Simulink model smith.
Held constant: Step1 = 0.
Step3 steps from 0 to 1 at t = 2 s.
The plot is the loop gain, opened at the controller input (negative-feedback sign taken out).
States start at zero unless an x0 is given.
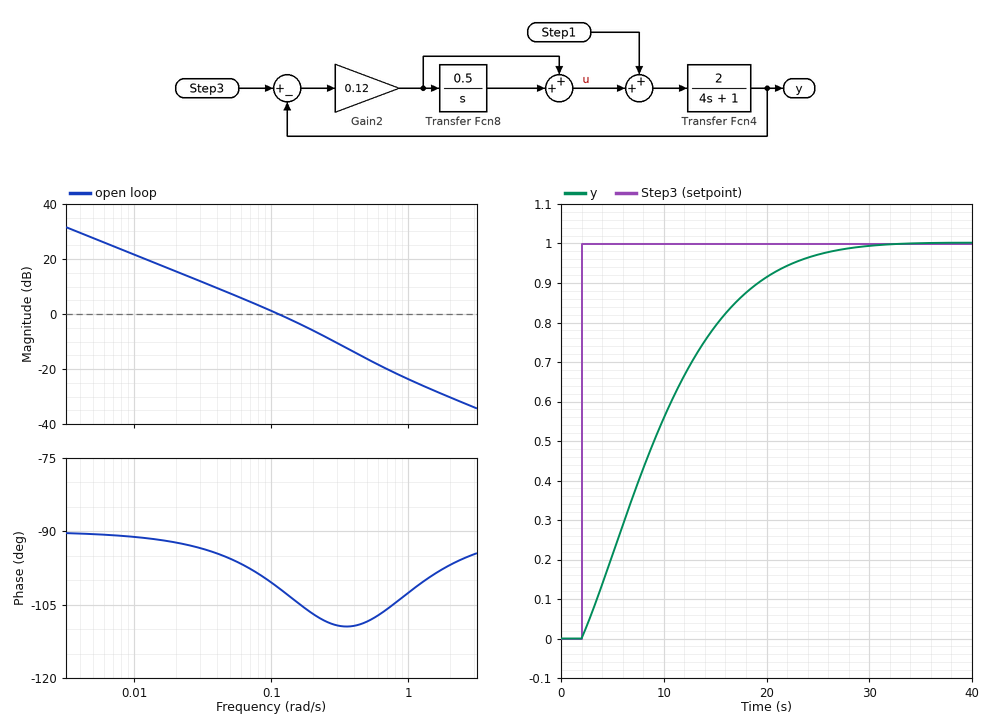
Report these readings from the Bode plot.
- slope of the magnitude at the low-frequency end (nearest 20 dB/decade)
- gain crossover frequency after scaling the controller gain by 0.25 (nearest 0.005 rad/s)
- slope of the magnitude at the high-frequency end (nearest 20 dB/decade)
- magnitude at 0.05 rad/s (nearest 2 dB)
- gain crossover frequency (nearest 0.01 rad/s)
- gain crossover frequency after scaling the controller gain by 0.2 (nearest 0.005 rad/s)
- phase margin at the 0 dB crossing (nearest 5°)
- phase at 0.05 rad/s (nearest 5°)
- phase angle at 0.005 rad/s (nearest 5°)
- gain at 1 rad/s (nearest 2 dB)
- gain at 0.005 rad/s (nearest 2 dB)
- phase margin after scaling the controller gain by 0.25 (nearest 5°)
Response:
-20 dB/decade
0.030 rad/s
-20 dB/decade
8 dB
0.11 rad/s
0.025 rad/s
80°
-95°
-90°
-24 dB
28 dB
85°
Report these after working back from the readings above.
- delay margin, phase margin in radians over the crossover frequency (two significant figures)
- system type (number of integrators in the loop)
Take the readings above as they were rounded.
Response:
13 s
1
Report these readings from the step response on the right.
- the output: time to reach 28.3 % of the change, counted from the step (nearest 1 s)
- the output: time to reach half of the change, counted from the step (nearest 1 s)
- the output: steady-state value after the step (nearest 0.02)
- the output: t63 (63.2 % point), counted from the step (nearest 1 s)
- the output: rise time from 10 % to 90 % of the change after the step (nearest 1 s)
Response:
4 s
7 s
1.00
9 s
16 s
